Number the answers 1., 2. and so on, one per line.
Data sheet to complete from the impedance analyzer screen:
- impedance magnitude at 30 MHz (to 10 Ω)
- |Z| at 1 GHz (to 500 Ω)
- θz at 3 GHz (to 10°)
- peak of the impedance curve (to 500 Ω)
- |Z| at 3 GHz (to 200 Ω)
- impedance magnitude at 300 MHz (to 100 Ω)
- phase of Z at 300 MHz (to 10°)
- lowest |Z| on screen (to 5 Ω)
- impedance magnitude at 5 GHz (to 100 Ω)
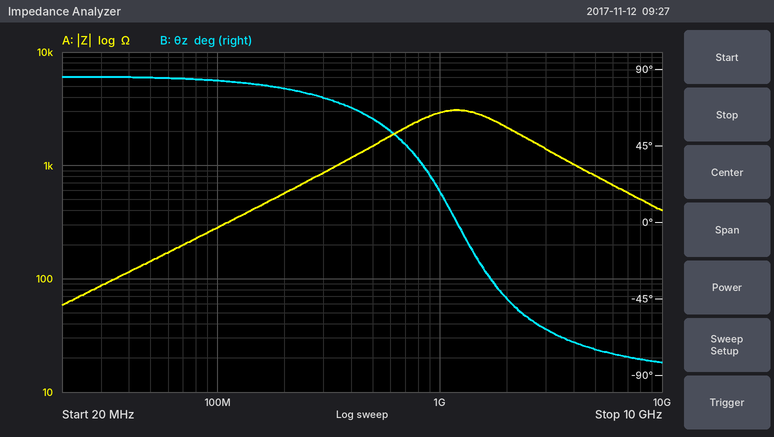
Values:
1. 90 Ω
2. 3.0 kΩ
3. -60°
4. 3.0 kΩ
5. 1.4 kΩ
6. 900 Ω
7. 70°
8. 60 Ω
9. 800 Ω
